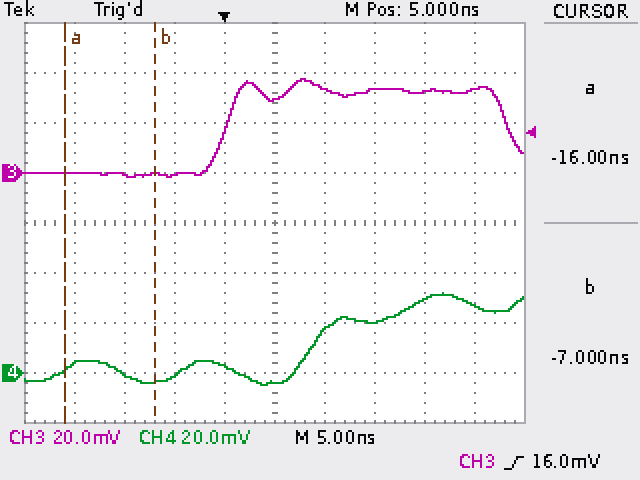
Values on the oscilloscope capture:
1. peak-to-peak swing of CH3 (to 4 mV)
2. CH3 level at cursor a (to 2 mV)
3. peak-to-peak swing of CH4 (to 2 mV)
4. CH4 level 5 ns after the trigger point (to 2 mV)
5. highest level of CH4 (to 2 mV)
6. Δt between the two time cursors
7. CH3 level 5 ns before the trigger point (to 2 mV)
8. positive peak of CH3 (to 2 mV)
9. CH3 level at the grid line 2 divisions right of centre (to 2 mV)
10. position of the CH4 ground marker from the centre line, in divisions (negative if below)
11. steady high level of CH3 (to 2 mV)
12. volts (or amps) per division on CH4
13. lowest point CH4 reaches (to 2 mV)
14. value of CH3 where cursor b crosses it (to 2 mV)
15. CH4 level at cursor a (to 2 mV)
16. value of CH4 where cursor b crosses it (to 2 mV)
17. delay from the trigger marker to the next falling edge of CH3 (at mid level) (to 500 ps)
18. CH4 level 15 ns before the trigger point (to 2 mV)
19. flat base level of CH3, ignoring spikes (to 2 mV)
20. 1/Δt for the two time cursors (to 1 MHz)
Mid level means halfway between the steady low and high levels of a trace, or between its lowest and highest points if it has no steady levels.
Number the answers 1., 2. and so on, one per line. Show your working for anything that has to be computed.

1. 40 mV
2. 0 mV
3. 32 mV − (-4 mV) = 36 mV
4. -4 mV
5. 32 mV
6. -7 ns − (-16 ns) = 9.0 ns
7. 0 mV
8. 38 mV
9. 34 mV
10. -3.0 div
11. 32 mV
12. 20 mV
13. -4 mV
14. 0 mV
15. 2 mV
16. -4 mV
17. 28.5 ns
18. 4 mV
19. 0 mV
20. 1 / 9.0 ns ≈ 111 MHz
